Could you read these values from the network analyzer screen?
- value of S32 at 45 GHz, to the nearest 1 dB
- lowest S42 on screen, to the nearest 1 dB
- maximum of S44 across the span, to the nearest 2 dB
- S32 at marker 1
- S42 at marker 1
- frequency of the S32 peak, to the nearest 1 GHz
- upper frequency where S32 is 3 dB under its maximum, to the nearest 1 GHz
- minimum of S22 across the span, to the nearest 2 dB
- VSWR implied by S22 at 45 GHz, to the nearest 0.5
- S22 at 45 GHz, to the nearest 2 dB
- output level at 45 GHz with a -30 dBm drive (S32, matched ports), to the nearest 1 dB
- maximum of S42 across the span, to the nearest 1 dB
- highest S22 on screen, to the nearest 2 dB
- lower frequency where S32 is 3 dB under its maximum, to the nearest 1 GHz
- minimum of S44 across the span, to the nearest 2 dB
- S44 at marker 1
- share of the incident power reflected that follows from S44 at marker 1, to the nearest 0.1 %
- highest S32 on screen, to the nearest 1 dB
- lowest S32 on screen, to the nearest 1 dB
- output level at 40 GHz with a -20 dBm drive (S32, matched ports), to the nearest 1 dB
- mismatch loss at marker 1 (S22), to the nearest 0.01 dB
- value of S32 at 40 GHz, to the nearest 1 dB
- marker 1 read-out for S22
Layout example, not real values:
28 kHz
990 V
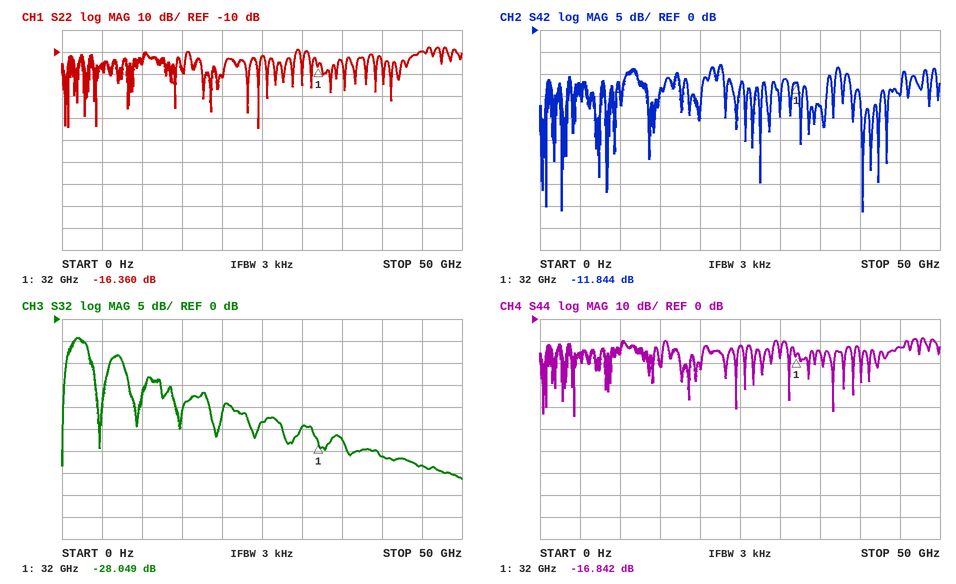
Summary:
-33 dB
-41 dB
-8 dB
-28.049 dB
-11.844 dB
2 GHz
3 GHz
-44 dB
2.0
-10 dB
-63 dBm
-8 dB
-8 dB
1 GHz
-44 dB
-16.842 dB
2.1 %
-4 dB
-36 dB
-51 dBm
0.10 dB
-31 dB
-16.360 dB
